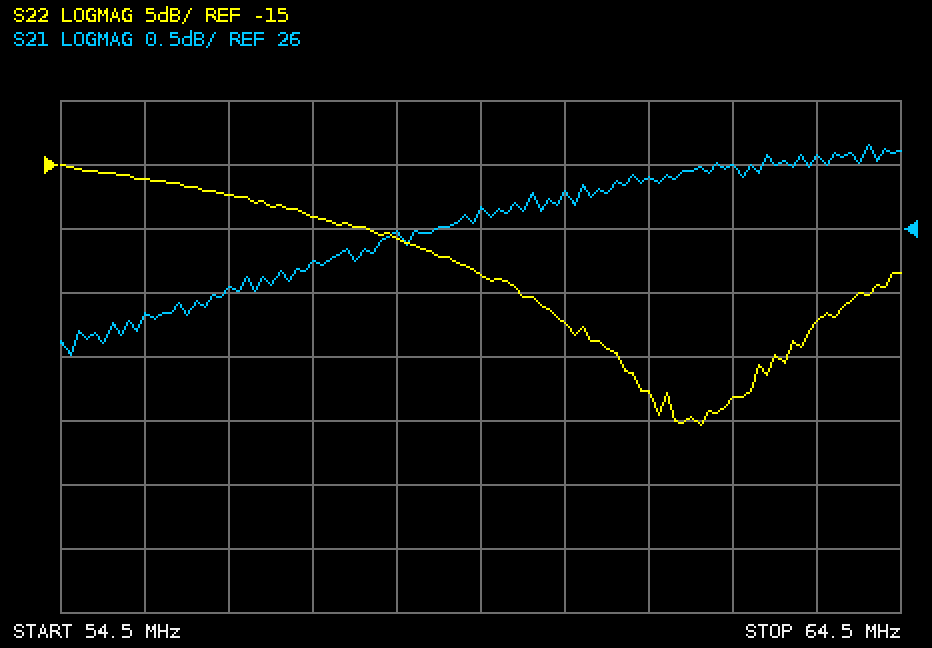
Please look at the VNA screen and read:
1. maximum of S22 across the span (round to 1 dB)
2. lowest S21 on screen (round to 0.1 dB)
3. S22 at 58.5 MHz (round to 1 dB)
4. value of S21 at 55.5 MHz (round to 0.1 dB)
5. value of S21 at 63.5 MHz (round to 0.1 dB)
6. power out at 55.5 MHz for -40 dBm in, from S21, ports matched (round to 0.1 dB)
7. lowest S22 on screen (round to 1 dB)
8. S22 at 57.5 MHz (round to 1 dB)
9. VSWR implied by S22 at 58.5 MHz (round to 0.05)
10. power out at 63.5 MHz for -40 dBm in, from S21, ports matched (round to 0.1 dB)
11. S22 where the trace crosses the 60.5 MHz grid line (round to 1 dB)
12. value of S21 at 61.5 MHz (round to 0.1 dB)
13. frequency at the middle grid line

-15 dB
25.0 dB
-21 dB
25.3 dB
26.6 dB
-14.7 dBm
-35 dB
-19 dB
1.20
-13.4 dBm
-27 dB
26.4 dB
59.5 MHz
